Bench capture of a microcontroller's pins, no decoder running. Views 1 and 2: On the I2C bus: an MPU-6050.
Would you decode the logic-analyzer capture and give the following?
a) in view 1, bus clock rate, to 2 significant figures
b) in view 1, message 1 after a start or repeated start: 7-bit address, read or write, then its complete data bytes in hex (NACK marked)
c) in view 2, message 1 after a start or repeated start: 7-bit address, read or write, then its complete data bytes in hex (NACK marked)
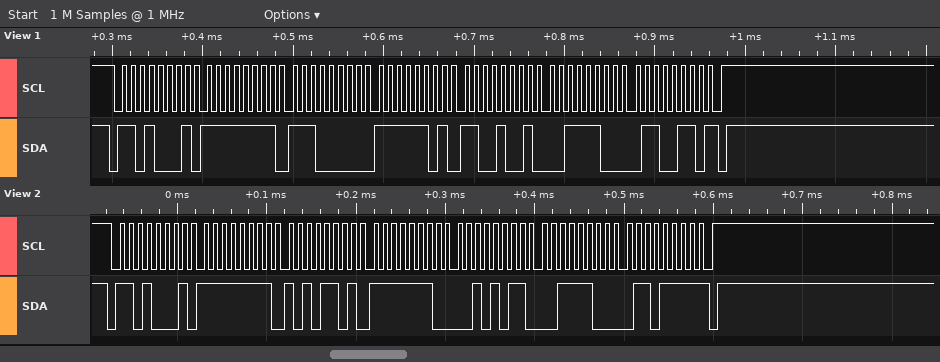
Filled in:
100 kHz
0x68 read: FF E0 FD C9 3C 66 NACK
0x68 read: FF AD FE 2B 3C 6F NACK
